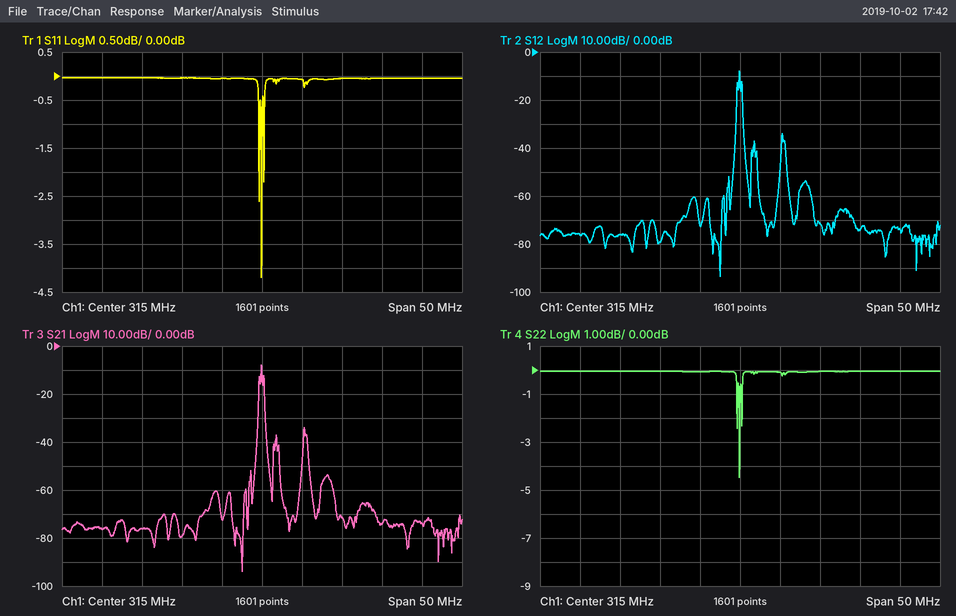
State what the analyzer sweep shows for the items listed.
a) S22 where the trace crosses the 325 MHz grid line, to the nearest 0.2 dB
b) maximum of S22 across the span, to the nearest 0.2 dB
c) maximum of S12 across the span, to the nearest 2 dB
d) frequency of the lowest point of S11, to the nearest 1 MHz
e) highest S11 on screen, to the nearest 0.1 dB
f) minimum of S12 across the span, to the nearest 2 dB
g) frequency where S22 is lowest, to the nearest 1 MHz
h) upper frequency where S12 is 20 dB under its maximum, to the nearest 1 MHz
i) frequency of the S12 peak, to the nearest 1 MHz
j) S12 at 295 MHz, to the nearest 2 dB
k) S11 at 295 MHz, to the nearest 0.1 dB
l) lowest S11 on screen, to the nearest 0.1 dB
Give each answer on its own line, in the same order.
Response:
0.0 dB
0.0 dB
-8 dB
315 MHz
0.0 dB
-94 dB
315 MHz
315 MHz
315 MHz
-76 dB
0.0 dB
-4.2 dB
